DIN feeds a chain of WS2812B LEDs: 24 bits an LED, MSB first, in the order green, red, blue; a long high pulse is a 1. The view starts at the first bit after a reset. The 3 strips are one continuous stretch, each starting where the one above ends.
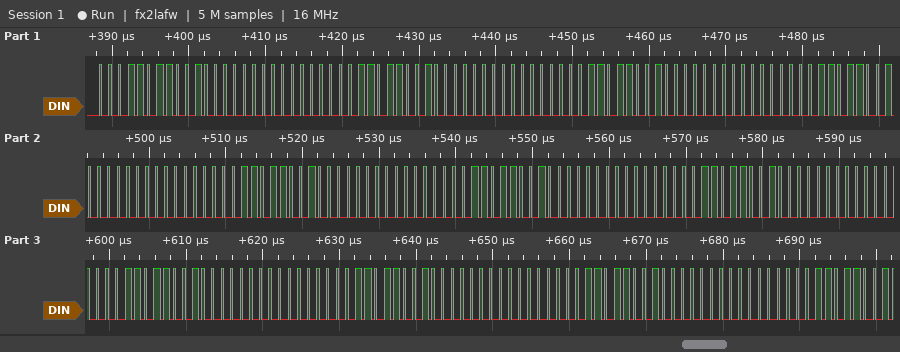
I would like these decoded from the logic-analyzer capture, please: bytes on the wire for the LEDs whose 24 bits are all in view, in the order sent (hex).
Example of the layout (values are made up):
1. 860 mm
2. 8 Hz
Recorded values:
1. 1B 20 00 1B 20 00 1B 20 00 1B 20 00 1B 20 00 1B 20 00 1B 20 00 1B 20 00 1B 20 00 1B 20 00
